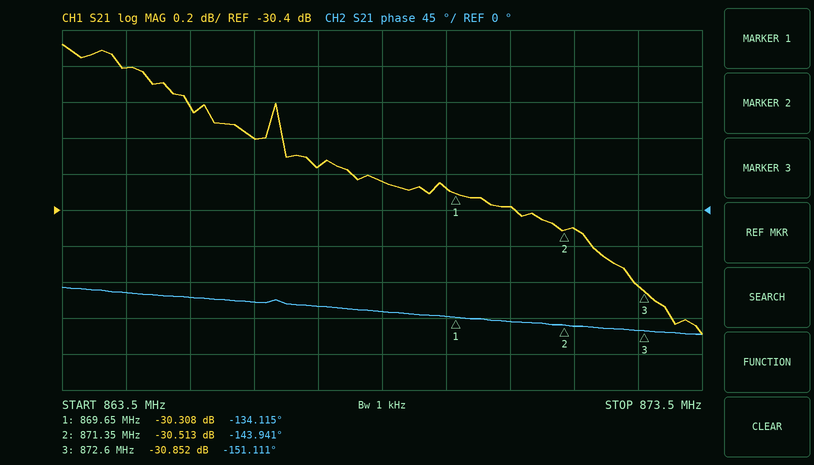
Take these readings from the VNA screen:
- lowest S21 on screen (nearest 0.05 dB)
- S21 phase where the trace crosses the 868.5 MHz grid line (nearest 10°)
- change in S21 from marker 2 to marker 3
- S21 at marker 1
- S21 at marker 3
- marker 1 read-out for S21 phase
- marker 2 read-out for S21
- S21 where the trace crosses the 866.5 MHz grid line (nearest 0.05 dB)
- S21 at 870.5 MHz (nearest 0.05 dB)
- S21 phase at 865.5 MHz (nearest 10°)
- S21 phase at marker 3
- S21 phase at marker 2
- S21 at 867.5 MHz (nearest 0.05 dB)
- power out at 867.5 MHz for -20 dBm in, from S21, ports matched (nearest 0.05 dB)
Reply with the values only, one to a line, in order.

-31.10 dB
-130°
-0.339 dB
-30.308 dB
-30.852 dB
-134.115°
-30.513 dB
-30.00 dB
-30.40 dB
-110°
-151.111°
-143.941°
-30.15 dB
-50.15 dBm
